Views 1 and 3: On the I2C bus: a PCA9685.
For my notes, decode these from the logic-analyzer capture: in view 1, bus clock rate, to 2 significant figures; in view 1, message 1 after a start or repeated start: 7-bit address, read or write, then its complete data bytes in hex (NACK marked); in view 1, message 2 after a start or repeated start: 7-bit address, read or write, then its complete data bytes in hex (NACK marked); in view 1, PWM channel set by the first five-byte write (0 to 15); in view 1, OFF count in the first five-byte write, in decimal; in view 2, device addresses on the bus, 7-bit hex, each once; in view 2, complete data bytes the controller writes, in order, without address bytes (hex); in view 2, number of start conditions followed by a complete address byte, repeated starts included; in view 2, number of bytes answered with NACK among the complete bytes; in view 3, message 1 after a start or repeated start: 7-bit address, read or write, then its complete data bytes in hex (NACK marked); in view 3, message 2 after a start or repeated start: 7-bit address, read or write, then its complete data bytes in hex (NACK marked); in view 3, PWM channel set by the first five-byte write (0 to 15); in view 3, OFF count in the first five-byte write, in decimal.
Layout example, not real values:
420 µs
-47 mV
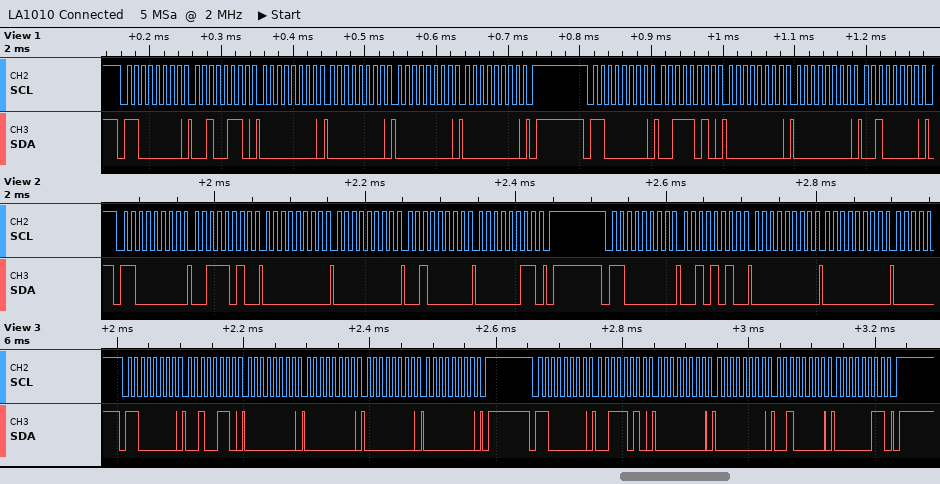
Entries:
100 kHz
0x60 write: 26 00 00 00 00
0x60 write: 3A 00 00 20
8
0
0x60
3A 00 00 20 03 2A 00 00
2
0
0x60 write: 26 00 00 00 00
0x60 write: 3A 00 00 20 03
8
0
